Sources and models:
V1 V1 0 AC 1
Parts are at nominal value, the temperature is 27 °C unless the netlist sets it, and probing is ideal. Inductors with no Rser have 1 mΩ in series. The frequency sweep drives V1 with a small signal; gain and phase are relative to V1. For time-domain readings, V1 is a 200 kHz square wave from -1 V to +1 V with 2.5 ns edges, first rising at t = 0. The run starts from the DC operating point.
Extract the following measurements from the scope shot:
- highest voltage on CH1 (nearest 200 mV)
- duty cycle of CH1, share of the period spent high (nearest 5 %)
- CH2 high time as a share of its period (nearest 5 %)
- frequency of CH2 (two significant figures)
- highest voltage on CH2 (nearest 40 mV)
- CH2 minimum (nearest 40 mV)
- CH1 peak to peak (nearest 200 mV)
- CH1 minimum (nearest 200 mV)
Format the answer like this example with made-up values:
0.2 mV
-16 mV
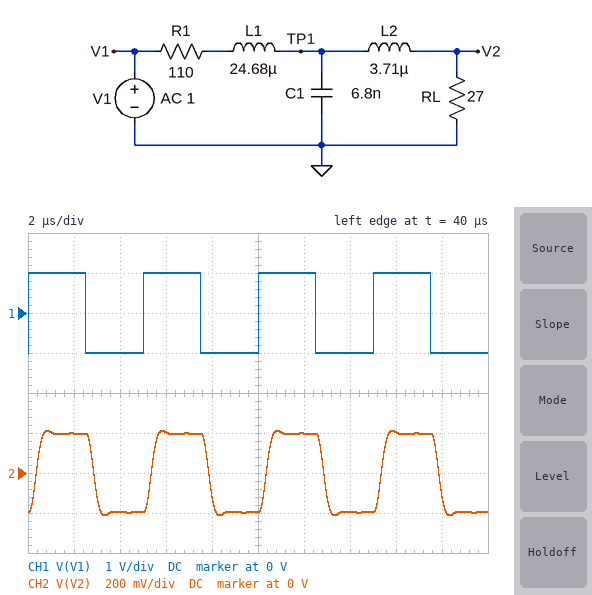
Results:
1.0 V
50 %
50 %
200 kHz
200 mV
-200 mV
2.0 V
-1.0 V
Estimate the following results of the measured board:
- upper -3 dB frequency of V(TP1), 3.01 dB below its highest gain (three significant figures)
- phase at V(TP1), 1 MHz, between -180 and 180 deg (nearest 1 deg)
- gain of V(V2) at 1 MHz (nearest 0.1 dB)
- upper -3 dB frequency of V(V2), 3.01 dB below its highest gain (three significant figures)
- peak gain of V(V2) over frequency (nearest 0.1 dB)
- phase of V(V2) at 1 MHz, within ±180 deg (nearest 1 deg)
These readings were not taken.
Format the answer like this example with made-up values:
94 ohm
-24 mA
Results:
1.15 MHz
-94 deg
-18.0 dB
923 kHz
-14.1 dB
-135 deg
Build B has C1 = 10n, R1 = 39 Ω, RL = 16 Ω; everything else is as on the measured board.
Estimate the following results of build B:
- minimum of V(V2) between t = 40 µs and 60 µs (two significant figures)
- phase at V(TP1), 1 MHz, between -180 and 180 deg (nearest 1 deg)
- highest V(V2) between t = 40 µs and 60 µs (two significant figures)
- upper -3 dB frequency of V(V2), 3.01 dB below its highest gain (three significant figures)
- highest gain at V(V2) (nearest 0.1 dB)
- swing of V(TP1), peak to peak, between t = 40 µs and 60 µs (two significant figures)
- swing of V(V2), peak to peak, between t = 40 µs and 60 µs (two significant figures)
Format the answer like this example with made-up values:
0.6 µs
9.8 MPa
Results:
-290 mV
-128 deg
290 mV
443 kHz
-10.7 dB
580 mV
570 mV
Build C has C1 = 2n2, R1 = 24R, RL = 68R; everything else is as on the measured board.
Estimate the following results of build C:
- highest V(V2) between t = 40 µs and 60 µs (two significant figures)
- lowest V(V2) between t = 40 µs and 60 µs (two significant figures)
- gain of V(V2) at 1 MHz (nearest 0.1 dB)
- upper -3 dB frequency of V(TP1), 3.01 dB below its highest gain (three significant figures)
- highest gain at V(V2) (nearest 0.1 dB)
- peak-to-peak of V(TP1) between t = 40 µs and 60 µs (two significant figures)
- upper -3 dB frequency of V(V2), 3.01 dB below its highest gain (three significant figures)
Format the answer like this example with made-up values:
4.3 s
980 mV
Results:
740 mV
-740 mV
-7.6 dB
796 kHz
-2.6 dB
1.5 V
753 kHz
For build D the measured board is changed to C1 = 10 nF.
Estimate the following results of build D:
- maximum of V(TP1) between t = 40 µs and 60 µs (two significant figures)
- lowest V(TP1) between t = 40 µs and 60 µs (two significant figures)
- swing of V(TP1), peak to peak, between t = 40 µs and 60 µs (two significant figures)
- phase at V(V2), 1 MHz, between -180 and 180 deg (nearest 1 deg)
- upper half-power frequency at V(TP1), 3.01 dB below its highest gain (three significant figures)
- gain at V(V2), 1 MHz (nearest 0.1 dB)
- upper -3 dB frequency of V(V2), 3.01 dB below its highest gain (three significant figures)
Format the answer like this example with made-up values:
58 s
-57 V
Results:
220 mV
-220 mV
430 mV
-154 deg
849 kHz
-21.4 dB
710 kHz
